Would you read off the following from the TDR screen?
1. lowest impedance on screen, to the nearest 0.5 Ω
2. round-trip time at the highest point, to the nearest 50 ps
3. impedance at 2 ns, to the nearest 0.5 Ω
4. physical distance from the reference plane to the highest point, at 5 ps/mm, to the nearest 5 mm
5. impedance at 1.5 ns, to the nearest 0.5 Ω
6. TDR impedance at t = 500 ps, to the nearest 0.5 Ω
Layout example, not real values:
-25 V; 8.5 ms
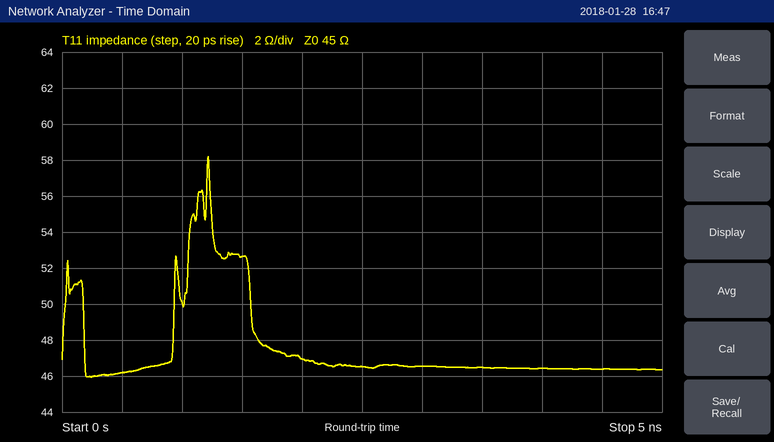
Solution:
46.0 Ω; 1.20 ns; 47.0 Ω; 120 mm; 52.5 Ω; 46.0 Ω
